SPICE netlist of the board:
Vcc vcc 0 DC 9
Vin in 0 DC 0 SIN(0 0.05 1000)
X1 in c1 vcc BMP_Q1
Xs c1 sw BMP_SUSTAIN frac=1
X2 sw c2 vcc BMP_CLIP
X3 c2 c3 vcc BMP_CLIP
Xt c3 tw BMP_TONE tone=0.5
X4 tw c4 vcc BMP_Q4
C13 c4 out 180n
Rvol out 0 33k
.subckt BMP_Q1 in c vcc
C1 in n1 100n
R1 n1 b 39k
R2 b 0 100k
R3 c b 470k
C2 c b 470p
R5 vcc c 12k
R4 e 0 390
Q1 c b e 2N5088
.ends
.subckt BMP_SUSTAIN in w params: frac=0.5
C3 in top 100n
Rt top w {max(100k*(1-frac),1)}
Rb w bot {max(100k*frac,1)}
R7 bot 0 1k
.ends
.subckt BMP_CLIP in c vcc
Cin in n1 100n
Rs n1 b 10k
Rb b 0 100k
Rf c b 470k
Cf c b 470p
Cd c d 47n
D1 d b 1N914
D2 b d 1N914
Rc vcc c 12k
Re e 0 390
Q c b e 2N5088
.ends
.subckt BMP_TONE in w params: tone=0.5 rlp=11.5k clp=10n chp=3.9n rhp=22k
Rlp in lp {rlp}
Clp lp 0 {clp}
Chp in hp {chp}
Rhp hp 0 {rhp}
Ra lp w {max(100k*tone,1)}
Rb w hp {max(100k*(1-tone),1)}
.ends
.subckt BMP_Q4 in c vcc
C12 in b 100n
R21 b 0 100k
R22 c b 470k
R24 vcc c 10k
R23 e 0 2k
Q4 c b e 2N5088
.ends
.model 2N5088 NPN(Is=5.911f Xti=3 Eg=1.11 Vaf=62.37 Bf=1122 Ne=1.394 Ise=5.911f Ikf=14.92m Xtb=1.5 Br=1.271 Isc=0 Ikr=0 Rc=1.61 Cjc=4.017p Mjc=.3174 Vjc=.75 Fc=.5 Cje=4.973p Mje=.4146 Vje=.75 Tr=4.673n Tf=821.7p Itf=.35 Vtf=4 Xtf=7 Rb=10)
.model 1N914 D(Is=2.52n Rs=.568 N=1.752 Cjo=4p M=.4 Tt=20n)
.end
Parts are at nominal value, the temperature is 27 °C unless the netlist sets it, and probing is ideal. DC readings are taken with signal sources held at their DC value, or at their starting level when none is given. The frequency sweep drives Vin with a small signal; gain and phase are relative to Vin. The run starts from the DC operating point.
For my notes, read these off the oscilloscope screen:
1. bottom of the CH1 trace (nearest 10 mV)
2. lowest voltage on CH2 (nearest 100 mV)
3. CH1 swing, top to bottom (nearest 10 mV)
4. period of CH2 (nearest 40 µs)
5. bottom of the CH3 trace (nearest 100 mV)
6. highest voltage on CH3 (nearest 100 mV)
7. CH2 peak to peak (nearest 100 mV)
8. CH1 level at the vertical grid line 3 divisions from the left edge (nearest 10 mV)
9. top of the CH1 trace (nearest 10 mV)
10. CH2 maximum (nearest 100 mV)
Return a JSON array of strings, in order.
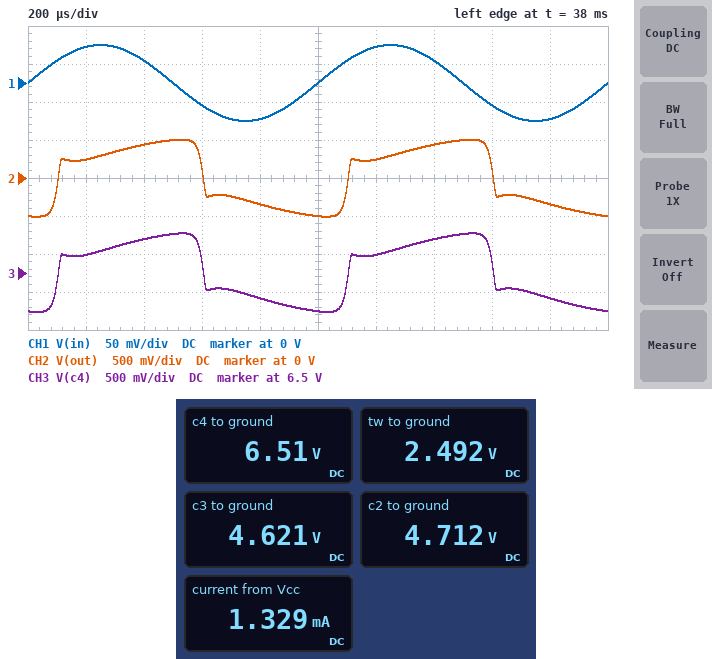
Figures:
["-50 mV", "-500 mV", "100 mV", "1.00 ms", "6.0 V", "7.0 V", "1.0 V", "-30 mV", "50 mV", "500 mV"]
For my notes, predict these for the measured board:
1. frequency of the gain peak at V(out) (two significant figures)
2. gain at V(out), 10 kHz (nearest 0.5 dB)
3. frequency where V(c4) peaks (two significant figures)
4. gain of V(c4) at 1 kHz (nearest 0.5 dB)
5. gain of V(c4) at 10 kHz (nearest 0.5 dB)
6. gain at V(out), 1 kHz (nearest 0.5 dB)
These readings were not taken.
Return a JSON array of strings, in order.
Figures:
["260 Hz", "15.5 dB", "250 Hz", "51.0 dB", "15.5 dB", "51.0 dB"]
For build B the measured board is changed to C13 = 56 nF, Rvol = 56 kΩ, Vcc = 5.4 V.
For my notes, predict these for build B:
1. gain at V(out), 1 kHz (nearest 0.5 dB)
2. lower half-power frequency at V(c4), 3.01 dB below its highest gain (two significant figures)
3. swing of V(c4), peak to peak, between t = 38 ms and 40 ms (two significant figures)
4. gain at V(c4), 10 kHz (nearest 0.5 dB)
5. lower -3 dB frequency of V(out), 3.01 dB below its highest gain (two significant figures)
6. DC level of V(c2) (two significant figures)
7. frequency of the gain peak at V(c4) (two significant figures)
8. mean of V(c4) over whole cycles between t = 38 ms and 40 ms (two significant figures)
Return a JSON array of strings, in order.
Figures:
["47.0 dB", "84 Hz", "950 mV", "14.0 dB", "97 Hz", "3.9 V", "240 Hz", "4.5 V"]
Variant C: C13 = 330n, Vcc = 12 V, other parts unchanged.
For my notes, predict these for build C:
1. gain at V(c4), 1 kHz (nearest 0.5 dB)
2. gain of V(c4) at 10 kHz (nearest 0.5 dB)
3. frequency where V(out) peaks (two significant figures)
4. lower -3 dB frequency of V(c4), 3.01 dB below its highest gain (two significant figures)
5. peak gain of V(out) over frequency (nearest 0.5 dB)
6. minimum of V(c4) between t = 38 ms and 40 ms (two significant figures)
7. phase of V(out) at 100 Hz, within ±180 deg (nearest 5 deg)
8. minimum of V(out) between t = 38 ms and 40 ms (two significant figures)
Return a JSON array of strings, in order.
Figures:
["52.0 dB", "16.0 dB", "260 Hz", "96 Hz", "58.0 dB", "7.6 V", "95 deg", "-530 mV"]
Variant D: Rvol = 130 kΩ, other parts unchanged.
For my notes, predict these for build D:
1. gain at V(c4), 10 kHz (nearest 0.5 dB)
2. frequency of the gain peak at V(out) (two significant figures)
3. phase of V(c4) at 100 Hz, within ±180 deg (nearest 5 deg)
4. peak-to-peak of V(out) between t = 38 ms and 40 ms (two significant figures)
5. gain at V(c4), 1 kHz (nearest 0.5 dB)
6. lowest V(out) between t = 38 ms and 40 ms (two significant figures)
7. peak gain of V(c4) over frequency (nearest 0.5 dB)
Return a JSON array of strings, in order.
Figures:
["17.0 dB", "250 Hz", "90 deg", "1.2 V", "52.5 dB", "-600 mV", "58.5 dB"]
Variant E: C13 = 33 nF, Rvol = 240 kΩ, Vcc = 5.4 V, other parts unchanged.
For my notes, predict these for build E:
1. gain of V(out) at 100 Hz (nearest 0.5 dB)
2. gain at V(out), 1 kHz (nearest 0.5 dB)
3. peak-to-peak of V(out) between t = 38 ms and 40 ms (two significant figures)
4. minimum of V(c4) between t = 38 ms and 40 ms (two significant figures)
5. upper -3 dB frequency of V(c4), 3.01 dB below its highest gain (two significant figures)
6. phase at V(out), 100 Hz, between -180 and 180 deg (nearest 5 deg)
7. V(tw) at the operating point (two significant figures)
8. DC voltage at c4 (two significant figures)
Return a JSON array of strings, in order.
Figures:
["51.5 dB", "48.0 dB", "1.0 V", "3.9 V", "710 Hz", "95 deg", "2.0 V", "4.5 V"]
